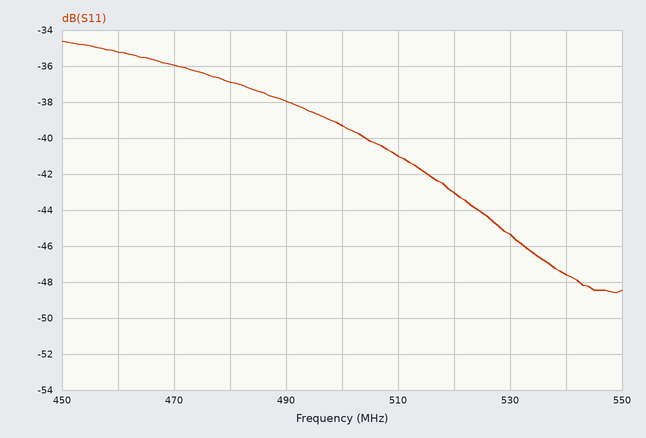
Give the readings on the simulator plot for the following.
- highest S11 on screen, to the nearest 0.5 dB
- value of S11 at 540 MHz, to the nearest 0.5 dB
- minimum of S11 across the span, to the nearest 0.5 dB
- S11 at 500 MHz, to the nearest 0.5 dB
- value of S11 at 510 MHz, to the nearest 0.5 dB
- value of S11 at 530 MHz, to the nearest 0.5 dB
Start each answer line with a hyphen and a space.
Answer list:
- -34.5 dB
- -47.5 dB
- -48.5 dB
- -39.5 dB
- -41.0 dB
- -45.5 dB
